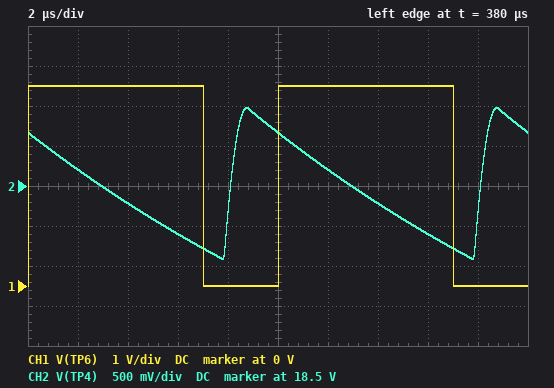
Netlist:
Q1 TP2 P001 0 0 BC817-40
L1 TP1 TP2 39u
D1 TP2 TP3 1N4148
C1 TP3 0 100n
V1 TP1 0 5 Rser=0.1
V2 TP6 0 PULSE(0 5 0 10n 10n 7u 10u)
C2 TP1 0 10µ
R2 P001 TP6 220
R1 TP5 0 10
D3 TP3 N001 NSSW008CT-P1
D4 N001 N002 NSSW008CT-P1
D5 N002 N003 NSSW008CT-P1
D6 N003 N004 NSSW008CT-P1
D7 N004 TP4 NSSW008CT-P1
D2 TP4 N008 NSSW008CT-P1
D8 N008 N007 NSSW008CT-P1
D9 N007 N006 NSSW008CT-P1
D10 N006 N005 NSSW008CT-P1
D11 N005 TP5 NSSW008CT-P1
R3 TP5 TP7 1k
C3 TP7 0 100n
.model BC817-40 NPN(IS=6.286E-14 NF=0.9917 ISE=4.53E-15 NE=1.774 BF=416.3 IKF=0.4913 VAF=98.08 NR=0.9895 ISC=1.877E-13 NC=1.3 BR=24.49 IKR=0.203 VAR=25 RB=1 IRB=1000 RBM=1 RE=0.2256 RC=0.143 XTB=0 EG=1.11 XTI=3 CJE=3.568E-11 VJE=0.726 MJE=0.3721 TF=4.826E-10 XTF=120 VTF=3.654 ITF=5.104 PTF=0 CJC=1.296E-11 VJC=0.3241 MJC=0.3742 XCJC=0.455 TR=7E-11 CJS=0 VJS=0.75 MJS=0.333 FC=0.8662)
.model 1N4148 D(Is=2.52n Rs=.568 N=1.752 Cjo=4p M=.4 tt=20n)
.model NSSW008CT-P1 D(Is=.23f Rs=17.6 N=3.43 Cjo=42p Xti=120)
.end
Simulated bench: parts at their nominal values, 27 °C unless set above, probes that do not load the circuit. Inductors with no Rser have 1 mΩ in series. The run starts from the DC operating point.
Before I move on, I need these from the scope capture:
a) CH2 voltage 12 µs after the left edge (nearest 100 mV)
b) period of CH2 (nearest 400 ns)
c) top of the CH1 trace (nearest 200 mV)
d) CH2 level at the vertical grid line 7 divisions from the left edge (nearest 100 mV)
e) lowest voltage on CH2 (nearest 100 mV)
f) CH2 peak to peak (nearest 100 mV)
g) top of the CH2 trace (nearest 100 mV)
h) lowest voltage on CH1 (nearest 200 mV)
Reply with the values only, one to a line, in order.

18.7 V
10.0 µs
5.0 V
18.3 V
17.6 V
1.9 V
19.5 V
0 V
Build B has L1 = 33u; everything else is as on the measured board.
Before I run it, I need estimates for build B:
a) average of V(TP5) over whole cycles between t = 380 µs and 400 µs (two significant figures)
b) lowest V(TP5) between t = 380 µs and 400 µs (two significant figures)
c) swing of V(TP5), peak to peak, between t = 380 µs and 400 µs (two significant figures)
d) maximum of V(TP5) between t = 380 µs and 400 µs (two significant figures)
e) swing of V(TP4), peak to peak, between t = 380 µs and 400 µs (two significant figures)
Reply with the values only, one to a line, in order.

440 mV
350 mV
190 mV
540 mV
2.1 V
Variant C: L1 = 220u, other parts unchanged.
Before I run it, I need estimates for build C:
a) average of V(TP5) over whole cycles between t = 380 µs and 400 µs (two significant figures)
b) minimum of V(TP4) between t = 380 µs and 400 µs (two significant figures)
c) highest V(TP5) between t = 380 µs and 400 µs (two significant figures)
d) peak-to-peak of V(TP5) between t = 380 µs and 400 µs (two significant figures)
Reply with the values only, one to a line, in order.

100 mV
15 V
120 mV
33 mV
